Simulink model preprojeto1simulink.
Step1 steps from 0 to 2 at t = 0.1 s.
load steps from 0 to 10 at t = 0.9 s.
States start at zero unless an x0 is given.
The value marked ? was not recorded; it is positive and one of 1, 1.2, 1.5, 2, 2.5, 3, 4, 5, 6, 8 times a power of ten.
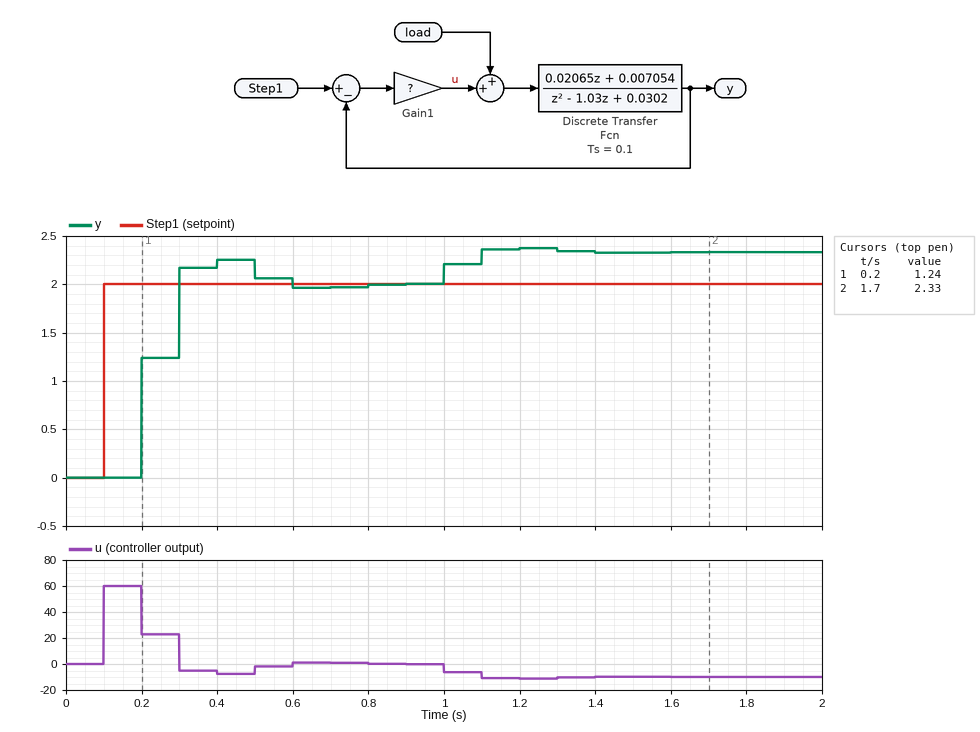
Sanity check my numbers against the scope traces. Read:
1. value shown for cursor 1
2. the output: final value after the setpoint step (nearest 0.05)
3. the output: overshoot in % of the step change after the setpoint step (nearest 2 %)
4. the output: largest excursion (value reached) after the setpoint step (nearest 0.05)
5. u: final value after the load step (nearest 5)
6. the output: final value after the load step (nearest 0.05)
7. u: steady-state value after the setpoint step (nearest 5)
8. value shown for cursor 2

1.24
2.00
12 %
2.25
-10
2.35
0
2.33
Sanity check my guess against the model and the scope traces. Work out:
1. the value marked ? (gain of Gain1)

30
